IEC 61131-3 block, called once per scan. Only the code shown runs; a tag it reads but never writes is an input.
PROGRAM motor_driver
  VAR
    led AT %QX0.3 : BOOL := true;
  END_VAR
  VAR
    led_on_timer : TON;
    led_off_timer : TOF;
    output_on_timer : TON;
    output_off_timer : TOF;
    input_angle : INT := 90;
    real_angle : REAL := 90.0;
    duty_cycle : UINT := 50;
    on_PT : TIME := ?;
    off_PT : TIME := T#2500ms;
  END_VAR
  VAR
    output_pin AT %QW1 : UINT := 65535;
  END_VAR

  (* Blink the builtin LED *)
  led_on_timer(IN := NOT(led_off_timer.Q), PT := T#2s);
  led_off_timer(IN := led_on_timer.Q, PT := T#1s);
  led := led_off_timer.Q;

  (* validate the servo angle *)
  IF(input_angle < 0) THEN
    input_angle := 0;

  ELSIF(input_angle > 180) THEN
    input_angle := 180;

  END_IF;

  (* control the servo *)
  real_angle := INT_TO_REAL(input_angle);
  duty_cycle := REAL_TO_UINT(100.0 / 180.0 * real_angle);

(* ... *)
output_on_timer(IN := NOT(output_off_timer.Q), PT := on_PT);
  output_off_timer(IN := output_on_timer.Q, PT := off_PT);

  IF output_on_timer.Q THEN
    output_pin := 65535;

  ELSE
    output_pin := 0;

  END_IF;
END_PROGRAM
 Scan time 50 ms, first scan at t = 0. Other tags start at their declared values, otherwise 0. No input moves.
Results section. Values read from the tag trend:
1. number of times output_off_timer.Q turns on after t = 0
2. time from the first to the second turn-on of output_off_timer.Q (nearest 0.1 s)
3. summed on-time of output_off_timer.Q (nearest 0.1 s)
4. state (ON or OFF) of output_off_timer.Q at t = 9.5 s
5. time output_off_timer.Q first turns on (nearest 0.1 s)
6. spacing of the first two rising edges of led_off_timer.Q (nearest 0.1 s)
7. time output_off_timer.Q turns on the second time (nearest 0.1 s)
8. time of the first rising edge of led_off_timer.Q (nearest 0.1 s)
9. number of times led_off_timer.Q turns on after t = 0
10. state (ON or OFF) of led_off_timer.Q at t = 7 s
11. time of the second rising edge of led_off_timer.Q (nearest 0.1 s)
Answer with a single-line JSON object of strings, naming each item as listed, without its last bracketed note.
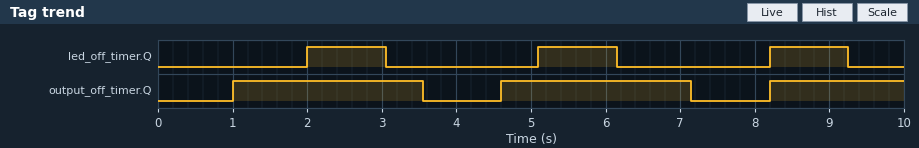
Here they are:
{"number of times output_off_timer.Q turns on after t = 0": "3", "time from the first to the second turn-on of output_off_timer.Q": "3.6 s", "summed on-time of output_off_timer.Q": "6.9 s", "state (ON or OFF) of output_off_timer.Q at t = 9.5 s": "ON", "time output_off_timer.Q first turns on": "1.0 s", "spacing of the first two rising edges of led_off_timer.Q": "3.1 s", "time output_off_timer.Q turns on the second time": "4.6 s", "time of the first rising edge of led_off_timer.Q": "2.0 s", "number of times led_off_timer.Q turns on after t = 0": "3", "state (ON or OFF) of led_off_timer.Q at t = 7 s": "OFF", "time of the second rising edge of led_off_timer.Q": "5.1 s"}
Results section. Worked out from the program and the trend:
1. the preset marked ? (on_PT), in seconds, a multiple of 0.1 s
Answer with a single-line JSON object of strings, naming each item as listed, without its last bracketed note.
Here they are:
{"the preset marked ? (on_PT), in seconds, a multiple of 0.1 s": "1.0 s"}
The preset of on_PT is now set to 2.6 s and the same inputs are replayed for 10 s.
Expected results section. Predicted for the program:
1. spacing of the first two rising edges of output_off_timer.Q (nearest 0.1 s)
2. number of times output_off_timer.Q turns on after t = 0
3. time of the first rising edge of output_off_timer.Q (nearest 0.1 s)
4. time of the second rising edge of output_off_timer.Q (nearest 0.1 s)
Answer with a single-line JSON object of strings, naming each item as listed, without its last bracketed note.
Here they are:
{"spacing of the first two rising edges of output_off_timer.Q": "5.2 s", "number of times output_off_timer.Q turns on after t = 0": "2", "time of the first rising edge of output_off_timer.Q": "2.6 s", "time of the second rising edge of output_off_timer.Q": "7.8 s"}
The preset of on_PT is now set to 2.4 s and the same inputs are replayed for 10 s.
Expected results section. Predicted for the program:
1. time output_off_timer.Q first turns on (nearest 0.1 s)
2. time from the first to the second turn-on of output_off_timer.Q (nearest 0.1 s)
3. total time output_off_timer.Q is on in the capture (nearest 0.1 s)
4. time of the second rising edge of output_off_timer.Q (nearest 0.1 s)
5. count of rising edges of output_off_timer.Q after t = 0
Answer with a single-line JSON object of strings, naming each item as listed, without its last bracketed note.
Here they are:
{"time output_off_timer.Q first turns on": "2.4 s", "time from the first to the second turn-on of output_off_timer.Q": "5.0 s", "total time output_off_timer.Q is on in the capture": "5.1 s", "time of the second rising edge of output_off_timer.Q": "7.4 s", "count of rising edges of output_off_timer.Q after t = 0": "2"}
